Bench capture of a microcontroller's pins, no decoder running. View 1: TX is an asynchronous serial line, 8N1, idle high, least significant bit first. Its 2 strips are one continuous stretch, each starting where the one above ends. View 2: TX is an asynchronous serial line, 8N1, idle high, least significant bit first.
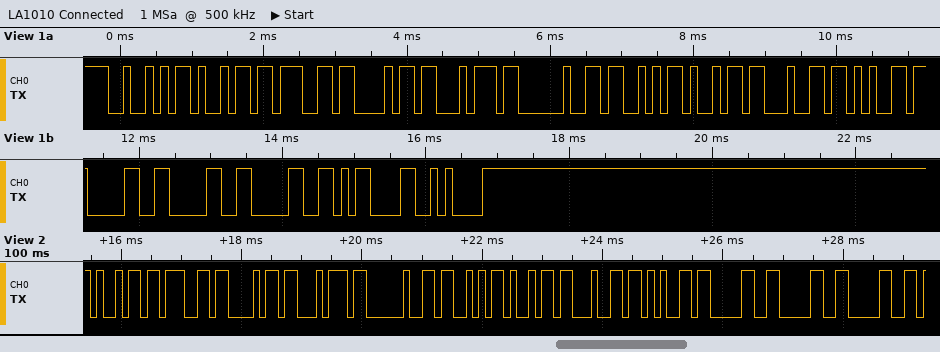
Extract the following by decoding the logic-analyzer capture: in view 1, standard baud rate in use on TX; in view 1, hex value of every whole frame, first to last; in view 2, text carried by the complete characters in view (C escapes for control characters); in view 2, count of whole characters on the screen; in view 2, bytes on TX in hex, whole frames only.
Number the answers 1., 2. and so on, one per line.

1. 9600 baud
2. 0x52 0x69 0x67 0x68 0x74 0x20 0x53 0x69 0x64 0x65 0x30 0x30 0x30 0x0D 0x0A
3. "ight Side000"
4. 12
5. 69 67 68 74 20 53 69 64 65 30 30 30
